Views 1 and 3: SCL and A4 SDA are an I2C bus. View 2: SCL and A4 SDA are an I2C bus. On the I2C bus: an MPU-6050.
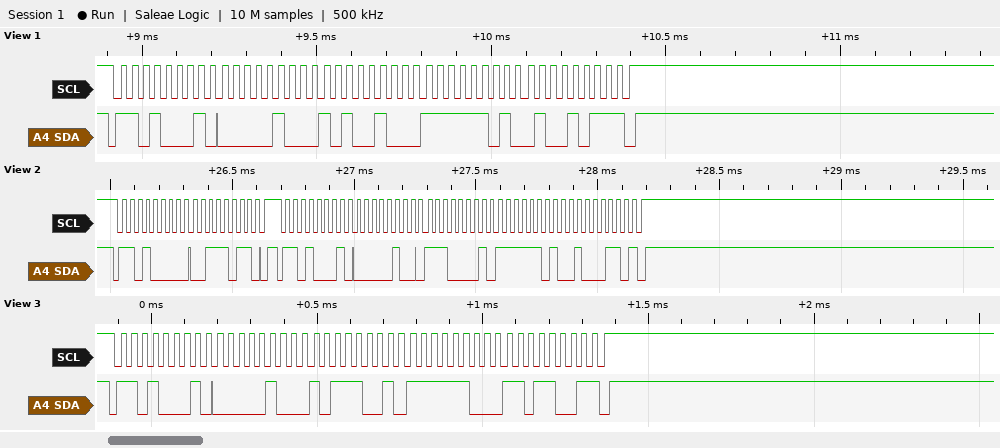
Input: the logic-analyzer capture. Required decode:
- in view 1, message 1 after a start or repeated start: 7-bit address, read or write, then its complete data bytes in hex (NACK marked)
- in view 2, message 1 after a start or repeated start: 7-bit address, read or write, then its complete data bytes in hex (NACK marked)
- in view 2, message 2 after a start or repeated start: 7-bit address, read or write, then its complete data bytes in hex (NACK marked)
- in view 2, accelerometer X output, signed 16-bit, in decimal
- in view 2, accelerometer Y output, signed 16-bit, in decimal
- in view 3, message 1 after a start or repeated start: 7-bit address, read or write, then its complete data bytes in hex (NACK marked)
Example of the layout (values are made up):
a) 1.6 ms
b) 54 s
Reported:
a) 0x68 read: 04 A4 FD 4B NACK
b) 0x68 write: 3B
c) 0x68 read: 04 E1 FD 46 NACK
d) 1249
e) -698
f) 0x68 read: 04 B9 FC D9 NACK
